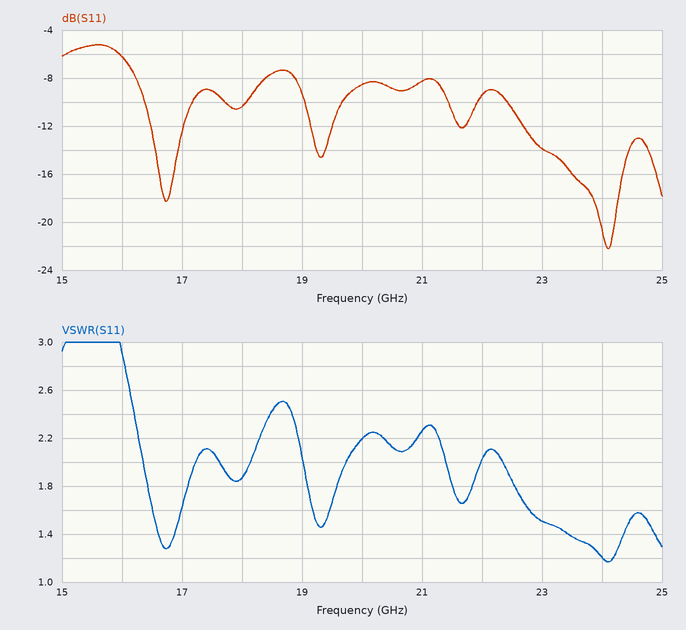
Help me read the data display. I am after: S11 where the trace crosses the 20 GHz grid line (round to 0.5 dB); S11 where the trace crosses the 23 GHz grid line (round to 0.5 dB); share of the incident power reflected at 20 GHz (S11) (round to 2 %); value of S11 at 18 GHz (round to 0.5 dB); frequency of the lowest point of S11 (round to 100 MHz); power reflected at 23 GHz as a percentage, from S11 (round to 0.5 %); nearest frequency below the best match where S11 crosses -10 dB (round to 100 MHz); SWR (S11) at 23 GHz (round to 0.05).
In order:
-8.5 dB
-14.0 dB
14 %
-10.5 dB
24.1 GHz
4.0 %
22.4 GHz
1.50
